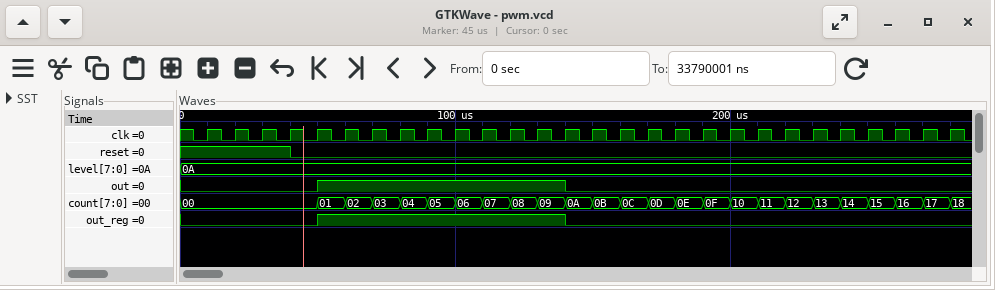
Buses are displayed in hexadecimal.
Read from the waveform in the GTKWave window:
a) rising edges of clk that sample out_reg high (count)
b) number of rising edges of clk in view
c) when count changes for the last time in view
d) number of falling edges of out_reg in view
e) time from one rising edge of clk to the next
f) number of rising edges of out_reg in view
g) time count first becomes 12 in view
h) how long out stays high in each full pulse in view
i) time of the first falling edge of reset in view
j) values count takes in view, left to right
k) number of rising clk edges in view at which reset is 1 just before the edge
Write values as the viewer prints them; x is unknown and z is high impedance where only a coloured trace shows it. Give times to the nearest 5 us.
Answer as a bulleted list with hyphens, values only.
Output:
- 9
- 28
- 280 us
- 1
- 10 us
- 1
- 220 us
- 90 us
- 40 us
- 00, 01, 02, 03, 04, 05, 06, 07, 08, 09, 0A, 0B, 0C, 0D, 0E, 0F, 10, 11, 12, 13, 14, 15, 16, 17, 18
- 4
